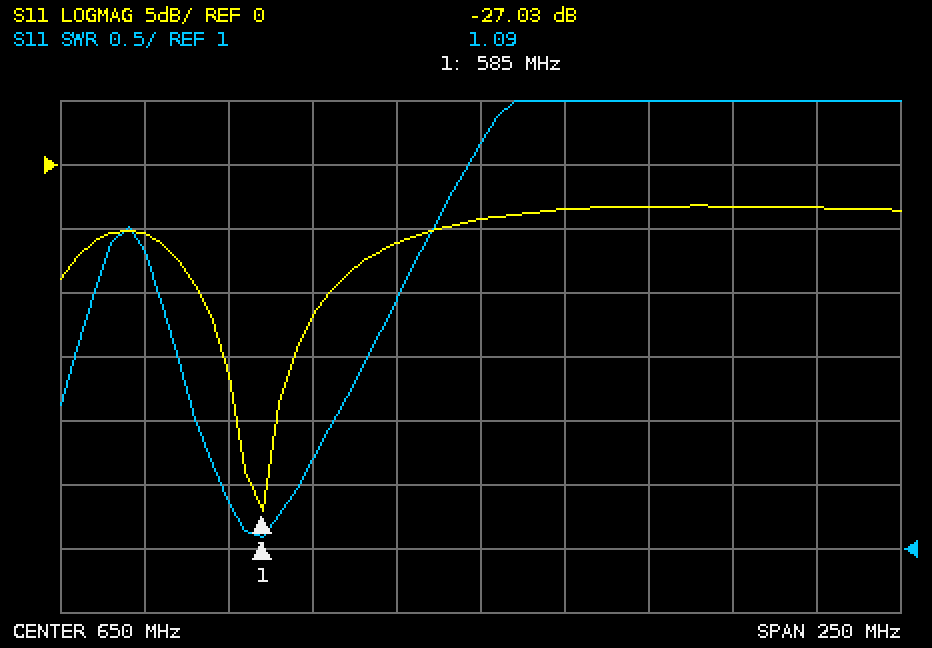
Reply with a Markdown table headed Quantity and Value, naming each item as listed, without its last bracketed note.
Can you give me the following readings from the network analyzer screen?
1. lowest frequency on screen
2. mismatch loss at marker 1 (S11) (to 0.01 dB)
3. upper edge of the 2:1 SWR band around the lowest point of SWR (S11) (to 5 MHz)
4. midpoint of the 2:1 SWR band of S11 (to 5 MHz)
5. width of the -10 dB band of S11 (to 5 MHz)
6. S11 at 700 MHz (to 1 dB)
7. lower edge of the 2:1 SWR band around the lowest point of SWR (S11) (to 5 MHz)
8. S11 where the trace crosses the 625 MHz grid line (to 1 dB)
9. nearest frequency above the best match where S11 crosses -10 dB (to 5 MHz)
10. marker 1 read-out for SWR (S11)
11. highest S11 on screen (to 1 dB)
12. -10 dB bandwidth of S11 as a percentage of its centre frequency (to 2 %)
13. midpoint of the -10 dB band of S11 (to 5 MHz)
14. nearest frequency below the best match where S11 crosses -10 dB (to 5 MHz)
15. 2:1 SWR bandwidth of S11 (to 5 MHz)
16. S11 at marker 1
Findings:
| Quantity | Value |
|---|---|
| lowest frequency on screen | 525 MHz |
| mismatch loss at marker 1 (S11) | 0.01 dB |
| upper edge of the 2:1 SWR band around the lowest point of SWR (S11) | 605 MHz |
| midpoint of the 2:1 SWR band of S11 | 585 MHz |
| width of the -10 dB band of S11 | 40 MHz |
| S11 at 700 MHz | -3 dB |
| lower edge of the 2:1 SWR band around the lowest point of SWR (S11) | 565 MHz |
| S11 where the trace crosses the 625 MHz grid line | -6 dB |
| nearest frequency above the best match where S11 crosses -10 dB | 605 MHz |
| marker 1 read-out for SWR | 1.09 |
| highest S11 on screen | -3 dB |
| -10 dB bandwidth of S11 as a percentage of its centre frequency | 6 % |
| midpoint of the -10 dB band of S11 | 585 MHz |
| nearest frequency below the best match where S11 crosses -10 dB | 565 MHz |
| 2:1 SWR bandwidth of S11 | 40 MHz |
| S11 at marker 1 | -27.03 dB |
